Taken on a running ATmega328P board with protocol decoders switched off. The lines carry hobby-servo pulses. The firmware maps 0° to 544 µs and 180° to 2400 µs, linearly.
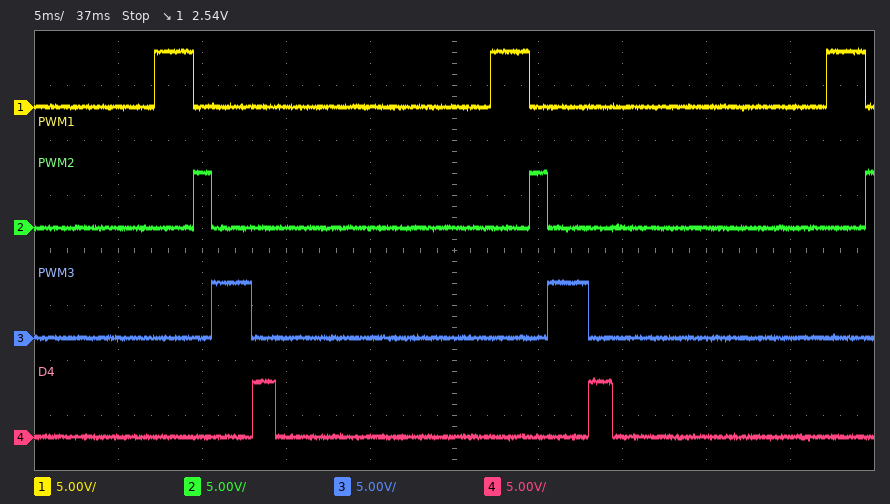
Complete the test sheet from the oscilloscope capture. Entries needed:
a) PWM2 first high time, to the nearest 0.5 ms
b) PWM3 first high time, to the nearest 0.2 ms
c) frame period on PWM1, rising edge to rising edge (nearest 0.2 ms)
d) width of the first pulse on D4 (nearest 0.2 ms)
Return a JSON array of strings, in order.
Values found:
["1.0 ms", "2.4 ms", "20.0 ms", "1.4 ms"]
